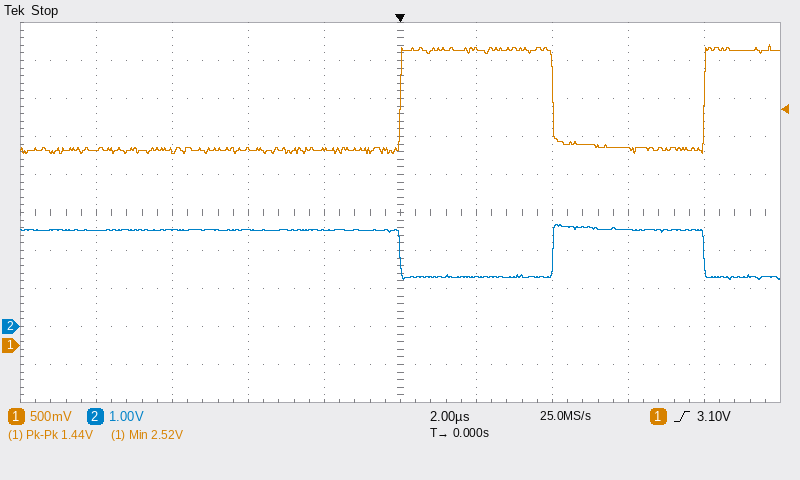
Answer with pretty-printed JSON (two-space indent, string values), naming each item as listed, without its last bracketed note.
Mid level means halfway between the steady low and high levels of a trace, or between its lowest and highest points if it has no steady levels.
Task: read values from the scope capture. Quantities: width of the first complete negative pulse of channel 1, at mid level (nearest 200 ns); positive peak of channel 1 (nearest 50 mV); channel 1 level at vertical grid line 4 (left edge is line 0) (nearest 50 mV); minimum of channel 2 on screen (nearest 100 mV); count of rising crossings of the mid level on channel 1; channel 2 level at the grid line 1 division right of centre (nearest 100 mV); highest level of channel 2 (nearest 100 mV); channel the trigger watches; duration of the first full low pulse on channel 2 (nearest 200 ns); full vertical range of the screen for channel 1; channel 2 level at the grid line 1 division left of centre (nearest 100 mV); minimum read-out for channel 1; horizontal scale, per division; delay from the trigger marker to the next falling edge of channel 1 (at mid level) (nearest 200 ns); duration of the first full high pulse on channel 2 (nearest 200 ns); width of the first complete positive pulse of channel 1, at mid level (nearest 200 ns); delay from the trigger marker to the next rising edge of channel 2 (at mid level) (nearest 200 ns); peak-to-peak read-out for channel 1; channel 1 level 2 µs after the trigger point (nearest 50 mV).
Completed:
{
  "width of the first complete negative pulse of channel 1, at mid level": "4.0 µs",
  "positive peak of channel 1": "3.95 V",
  "channel 1 level at vertical grid line 4 (left edge is line 0)": "2.60 V",
  "minimum of channel 2 on screen": "1.2 V",
  "count of rising crossings of the mid level on channel 1": "2",
  "channel 2 level at the grid line 1 division right of centre": "1.3 V",
  "highest level of channel 2": "2.7 V",
  "channel the trigger watches": "channel 1",
  "duration of the first full low pulse on channel 2": "4.0 µs",
  "full vertical range of the screen for channel 1": "5 V",
  "channel 2 level at the grid line 1 division left of centre": "2.5 V",
  "minimum read-out for channel 1": "2.52 V",
  "horizontal scale, per division": "2 µs",
  "delay from the trigger marker to the next falling edge of channel 1 (at mid level)": "4.0 µs",
  "duration of the first full high pulse on channel 2": "4.0 µs",
  "width of the first complete positive pulse of channel 1, at mid level": "4.0 µs",
  "delay from the trigger marker to the next rising edge of channel 2 (at mid level)": "4.0 µs",
  "peak-to-peak read-out for channel 1": "1.44 V",
  "channel 1 level 2 µs after the trigger point": "3.90 V"
}
